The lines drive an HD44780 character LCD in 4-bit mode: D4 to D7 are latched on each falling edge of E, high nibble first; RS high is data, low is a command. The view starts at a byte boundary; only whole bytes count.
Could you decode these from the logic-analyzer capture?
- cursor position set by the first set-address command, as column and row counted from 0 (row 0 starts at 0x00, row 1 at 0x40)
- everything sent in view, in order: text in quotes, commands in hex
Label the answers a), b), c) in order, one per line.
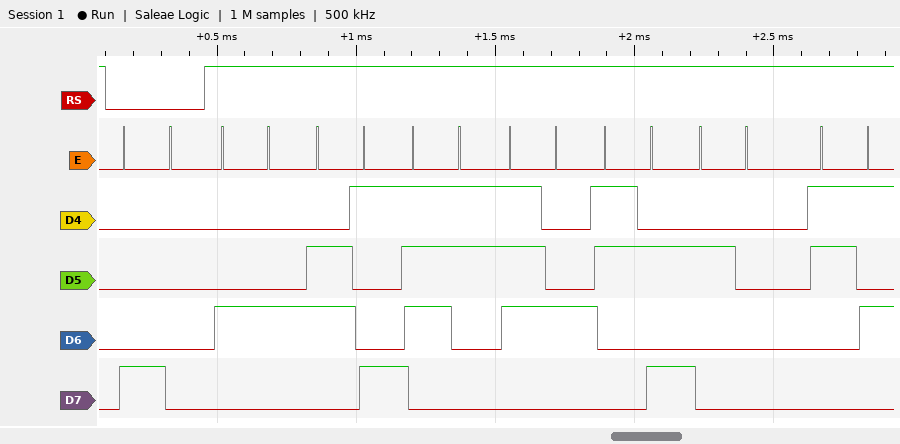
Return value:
a) column 0, row 0
b) 0x80 "Dist: 5"
